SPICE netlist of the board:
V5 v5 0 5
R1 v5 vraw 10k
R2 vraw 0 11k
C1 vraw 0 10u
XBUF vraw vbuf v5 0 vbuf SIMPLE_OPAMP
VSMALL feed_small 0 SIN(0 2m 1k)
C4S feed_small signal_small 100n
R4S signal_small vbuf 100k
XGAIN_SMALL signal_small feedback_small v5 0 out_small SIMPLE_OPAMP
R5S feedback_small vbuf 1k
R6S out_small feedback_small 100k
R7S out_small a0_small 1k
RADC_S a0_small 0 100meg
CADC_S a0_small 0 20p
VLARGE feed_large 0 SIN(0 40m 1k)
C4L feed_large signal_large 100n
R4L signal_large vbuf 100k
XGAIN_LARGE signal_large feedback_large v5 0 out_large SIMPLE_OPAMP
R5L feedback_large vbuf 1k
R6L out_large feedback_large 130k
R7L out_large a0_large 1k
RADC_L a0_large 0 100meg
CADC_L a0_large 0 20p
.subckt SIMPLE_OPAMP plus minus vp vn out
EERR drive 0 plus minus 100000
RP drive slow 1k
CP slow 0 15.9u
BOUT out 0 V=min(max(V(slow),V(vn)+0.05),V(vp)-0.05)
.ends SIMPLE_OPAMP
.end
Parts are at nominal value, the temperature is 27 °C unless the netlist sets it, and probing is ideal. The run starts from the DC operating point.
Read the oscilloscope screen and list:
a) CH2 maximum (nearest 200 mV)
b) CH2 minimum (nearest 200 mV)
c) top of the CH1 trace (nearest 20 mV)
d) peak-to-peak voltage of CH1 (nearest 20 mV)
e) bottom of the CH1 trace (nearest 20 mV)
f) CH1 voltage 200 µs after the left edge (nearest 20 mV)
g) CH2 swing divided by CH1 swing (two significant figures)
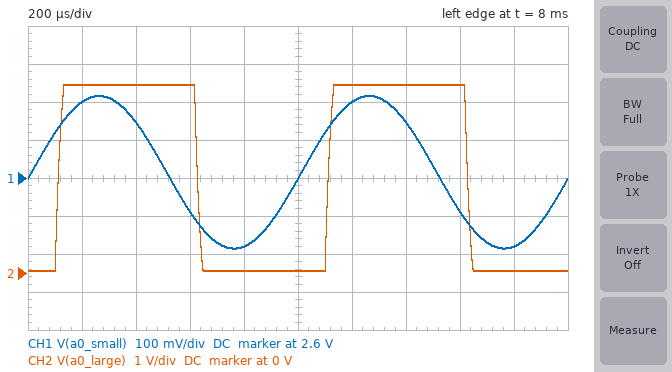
5.0 V
0 V
2.82 V
400 mV
2.42 V
2.80 V
12
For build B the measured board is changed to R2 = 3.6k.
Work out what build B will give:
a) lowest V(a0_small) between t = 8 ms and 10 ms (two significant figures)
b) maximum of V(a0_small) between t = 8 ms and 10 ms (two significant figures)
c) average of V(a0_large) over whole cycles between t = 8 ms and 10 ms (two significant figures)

1.1 V
1.5 V
1.3 V
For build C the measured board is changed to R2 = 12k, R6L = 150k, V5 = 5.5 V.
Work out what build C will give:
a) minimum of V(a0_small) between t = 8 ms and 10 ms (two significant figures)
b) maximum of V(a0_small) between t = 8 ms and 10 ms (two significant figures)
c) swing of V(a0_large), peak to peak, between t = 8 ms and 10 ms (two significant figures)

2.8 V
3.2 V
5.4 V
